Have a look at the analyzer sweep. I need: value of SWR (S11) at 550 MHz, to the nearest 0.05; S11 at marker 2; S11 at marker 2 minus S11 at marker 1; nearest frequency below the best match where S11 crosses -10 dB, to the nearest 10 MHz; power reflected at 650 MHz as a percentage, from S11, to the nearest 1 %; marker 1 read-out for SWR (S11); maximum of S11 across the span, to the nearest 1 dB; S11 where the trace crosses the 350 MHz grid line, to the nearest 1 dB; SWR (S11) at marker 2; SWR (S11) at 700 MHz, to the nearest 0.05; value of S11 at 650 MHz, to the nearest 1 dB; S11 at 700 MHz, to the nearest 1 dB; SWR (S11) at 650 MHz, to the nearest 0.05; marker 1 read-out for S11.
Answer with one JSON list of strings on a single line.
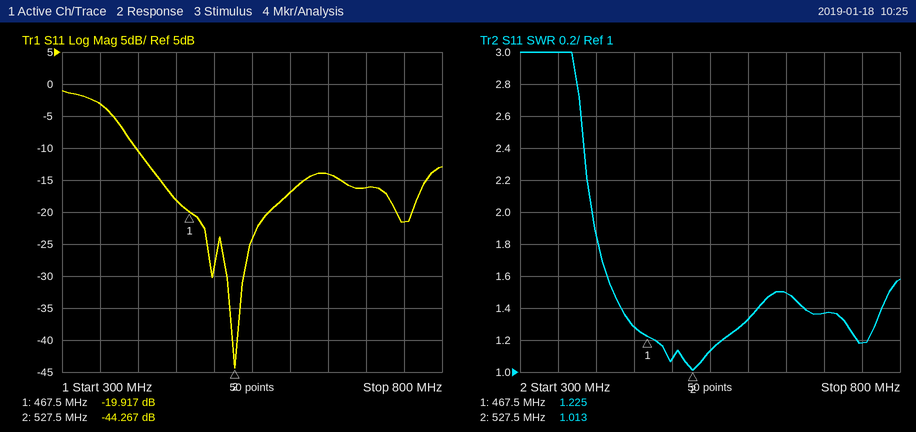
["1.15", "-44.267 dB", "-24.350 dB", "400 MHz", "4 %", "1.225", "-1 dB", "-3 dB", "1.013", "1.35", "-14 dB", "-16 dB", "1.50", "-19.917 dB"]
